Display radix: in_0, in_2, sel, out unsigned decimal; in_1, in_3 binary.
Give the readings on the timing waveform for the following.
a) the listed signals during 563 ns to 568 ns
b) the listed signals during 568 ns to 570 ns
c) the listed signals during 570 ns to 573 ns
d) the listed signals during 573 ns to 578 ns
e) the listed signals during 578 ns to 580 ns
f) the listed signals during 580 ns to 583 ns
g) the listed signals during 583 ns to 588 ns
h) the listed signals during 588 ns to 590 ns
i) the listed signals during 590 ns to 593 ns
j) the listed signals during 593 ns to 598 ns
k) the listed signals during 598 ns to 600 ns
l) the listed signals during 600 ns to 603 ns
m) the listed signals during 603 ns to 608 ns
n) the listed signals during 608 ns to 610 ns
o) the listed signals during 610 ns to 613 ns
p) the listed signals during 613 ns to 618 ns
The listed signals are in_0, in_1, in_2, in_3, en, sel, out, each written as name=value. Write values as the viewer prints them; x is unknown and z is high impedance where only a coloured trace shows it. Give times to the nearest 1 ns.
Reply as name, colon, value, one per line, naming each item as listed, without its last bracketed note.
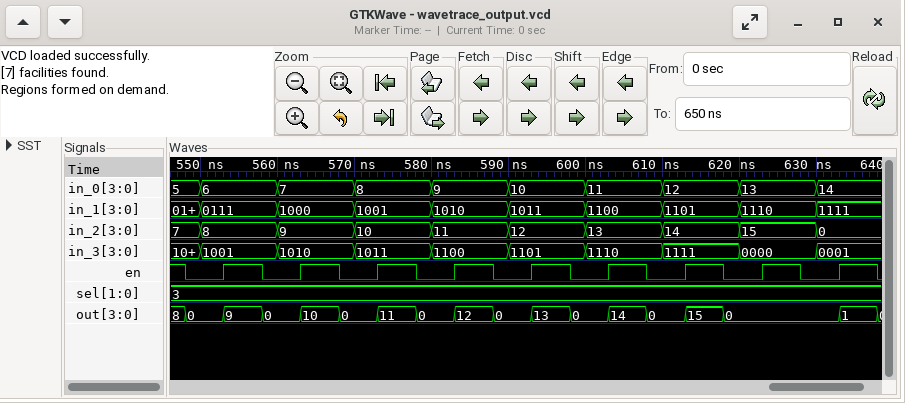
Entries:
the listed signals during 563 ns to 568 ns: in_0=7, in_1=1000, in_2=9, in_3=1010, en=1, sel=3, out=10
the listed signals during 568 ns to 570 ns: in_0=7, in_1=1000, in_2=9, in_3=1010, en=0, sel=3, out=0
the listed signals during 570 ns to 573 ns: in_0=8, in_1=1001, in_2=10, in_3=1011, en=0, sel=3, out=0
the listed signals during 573 ns to 578 ns: in_0=8, in_1=1001, in_2=10, in_3=1011, en=1, sel=3, out=11
the listed signals during 578 ns to 580 ns: in_0=8, in_1=1001, in_2=10, in_3=1011, en=0, sel=3, out=0
the listed signals during 580 ns to 583 ns: in_0=9, in_1=1010, in_2=11, in_3=1100, en=0, sel=3, out=0
the listed signals during 583 ns to 588 ns: in_0=9, in_1=1010, in_2=11, in_3=1100, en=1, sel=3, out=12
the listed signals during 588 ns to 590 ns: in_0=9, in_1=1010, in_2=11, in_3=1100, en=0, sel=3, out=0
the listed signals during 590 ns to 593 ns: in_0=10, in_1=1011, in_2=12, in_3=1101, en=0, sel=3, out=0
the listed signals during 593 ns to 598 ns: in_0=10, in_1=1011, in_2=12, in_3=1101, en=1, sel=3, out=13
the listed signals during 598 ns to 600 ns: in_0=10, in_1=1011, in_2=12, in_3=1101, en=0, sel=3, out=0
the listed signals during 600 ns to 603 ns: in_0=11, in_1=1100, in_2=13, in_3=1110, en=0, sel=3, out=0
the listed signals during 603 ns to 608 ns: in_0=11, in_1=1100, in_2=13, in_3=1110, en=1, sel=3, out=14
the listed signals during 608 ns to 610 ns: in_0=11, in_1=1100, in_2=13, in_3=1110, en=0, sel=3, out=0
the listed signals during 610 ns to 613 ns: in_0=12, in_1=1101, in_2=14, in_3=1111, en=0, sel=3, out=0
the listed signals during 613 ns to 618 ns: in_0=12, in_1=1101, in_2=14, in_3=1111, en=1, sel=3, out=15
